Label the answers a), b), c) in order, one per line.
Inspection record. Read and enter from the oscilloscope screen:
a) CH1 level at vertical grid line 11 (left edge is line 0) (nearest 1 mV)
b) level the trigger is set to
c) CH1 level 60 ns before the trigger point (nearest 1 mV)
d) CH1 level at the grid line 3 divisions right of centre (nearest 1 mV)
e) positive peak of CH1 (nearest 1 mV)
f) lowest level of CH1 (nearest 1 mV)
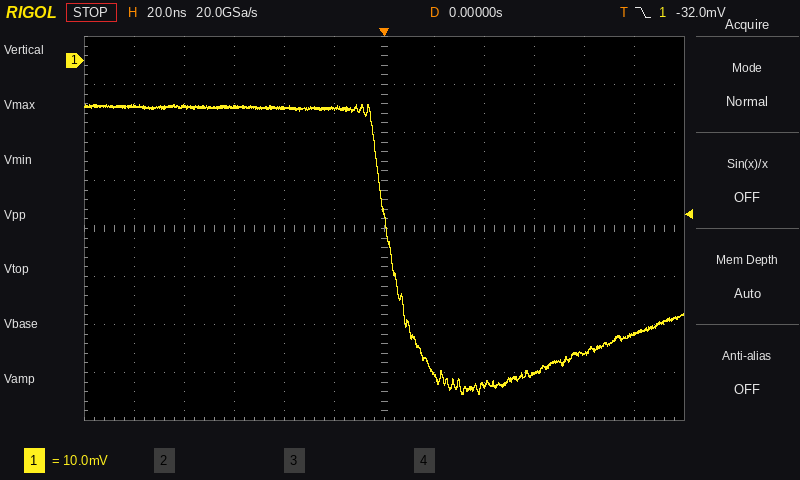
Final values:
a) -57 mV
b) -32.0 mV
c) -10 mV
d) -65 mV
e) -9 mV
f) -70 mV
